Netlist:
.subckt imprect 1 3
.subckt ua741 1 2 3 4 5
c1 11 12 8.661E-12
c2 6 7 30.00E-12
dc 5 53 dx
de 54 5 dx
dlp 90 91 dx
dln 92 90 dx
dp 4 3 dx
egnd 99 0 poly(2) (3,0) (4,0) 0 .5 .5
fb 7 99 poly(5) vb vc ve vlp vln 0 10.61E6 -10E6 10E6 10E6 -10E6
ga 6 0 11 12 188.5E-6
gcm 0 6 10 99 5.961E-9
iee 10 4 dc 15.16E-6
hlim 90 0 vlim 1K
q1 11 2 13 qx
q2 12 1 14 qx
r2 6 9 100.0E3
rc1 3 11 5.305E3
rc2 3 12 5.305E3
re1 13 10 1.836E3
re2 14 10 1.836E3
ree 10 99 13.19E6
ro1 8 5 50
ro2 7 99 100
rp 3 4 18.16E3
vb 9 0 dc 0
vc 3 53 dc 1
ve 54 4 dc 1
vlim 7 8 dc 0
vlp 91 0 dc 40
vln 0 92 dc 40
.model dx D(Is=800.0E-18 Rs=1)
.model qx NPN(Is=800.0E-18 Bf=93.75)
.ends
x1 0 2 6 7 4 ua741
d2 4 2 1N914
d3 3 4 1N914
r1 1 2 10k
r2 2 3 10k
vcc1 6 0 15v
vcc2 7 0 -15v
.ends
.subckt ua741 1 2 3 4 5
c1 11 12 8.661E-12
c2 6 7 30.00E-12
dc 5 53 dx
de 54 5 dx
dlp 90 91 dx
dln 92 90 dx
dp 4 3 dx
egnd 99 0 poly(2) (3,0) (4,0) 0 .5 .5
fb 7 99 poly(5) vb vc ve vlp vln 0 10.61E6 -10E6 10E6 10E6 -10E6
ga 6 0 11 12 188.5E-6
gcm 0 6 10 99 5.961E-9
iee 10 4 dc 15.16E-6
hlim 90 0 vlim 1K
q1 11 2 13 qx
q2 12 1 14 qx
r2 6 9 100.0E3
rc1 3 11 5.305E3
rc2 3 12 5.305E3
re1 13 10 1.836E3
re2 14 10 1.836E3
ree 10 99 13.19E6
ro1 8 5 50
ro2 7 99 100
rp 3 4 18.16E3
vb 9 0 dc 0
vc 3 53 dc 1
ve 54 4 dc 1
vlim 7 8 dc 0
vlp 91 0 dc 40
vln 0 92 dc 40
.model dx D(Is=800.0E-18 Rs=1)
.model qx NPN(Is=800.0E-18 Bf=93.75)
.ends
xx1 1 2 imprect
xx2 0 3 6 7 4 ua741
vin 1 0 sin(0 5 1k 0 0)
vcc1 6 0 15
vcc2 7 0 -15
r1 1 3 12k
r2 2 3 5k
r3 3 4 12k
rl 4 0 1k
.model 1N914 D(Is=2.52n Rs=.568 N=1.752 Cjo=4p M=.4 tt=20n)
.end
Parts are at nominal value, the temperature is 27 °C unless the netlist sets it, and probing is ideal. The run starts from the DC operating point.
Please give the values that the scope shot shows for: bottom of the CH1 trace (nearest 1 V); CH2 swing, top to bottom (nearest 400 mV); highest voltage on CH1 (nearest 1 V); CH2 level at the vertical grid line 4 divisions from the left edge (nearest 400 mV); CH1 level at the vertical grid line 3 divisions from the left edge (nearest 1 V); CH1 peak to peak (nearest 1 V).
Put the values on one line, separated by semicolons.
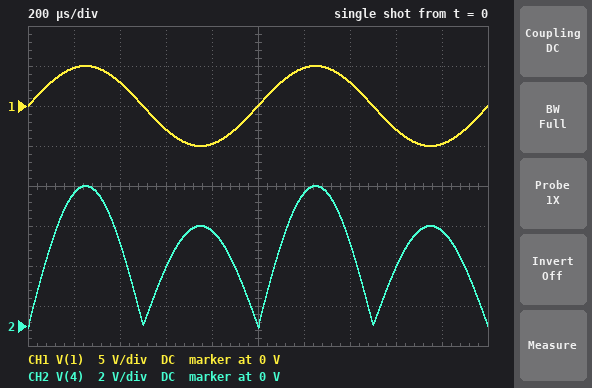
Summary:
-5 V; 7.2 V; 5 V; 4.8 V; -3 V; 10 V
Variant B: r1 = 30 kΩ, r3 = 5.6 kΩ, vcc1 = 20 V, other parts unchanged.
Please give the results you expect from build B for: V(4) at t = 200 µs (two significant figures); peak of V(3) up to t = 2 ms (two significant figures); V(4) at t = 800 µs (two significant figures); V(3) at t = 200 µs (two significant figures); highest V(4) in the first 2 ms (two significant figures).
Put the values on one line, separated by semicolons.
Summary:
4.4 V; 5.1 mV; 890 mV; -1.5 mV; 4.7 V
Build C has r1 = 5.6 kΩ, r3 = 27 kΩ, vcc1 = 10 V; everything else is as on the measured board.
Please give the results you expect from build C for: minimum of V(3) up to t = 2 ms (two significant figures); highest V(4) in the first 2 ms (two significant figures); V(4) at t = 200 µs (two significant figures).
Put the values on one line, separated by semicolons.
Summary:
-1.9 V; 9.6 V; 2.7 V
